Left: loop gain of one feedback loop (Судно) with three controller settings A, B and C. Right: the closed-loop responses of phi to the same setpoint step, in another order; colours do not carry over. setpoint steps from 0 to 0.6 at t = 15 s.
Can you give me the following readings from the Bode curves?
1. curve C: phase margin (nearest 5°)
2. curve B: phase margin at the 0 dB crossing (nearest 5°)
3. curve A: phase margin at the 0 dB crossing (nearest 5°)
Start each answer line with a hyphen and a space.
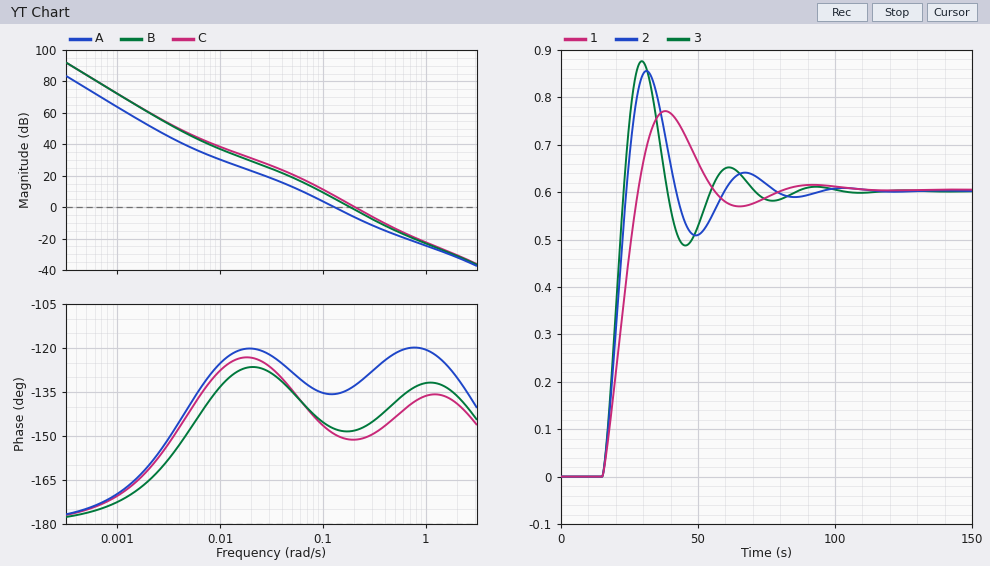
- 30°
- 30°
- 45°
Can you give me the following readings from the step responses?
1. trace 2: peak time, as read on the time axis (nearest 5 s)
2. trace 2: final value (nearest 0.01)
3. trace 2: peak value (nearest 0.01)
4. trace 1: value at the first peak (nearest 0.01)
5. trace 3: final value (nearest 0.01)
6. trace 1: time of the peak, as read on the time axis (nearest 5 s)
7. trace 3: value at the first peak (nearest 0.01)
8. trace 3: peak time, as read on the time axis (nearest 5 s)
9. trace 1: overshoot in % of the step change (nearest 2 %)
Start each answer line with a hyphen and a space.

- 30 s
- 0.60
- 0.86
- 0.77
- 0.60
- 40 s
- 0.88
- 30 s
- 28 %
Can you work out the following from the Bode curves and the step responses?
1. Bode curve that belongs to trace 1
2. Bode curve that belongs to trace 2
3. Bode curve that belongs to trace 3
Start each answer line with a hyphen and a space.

- A
- B
- C
